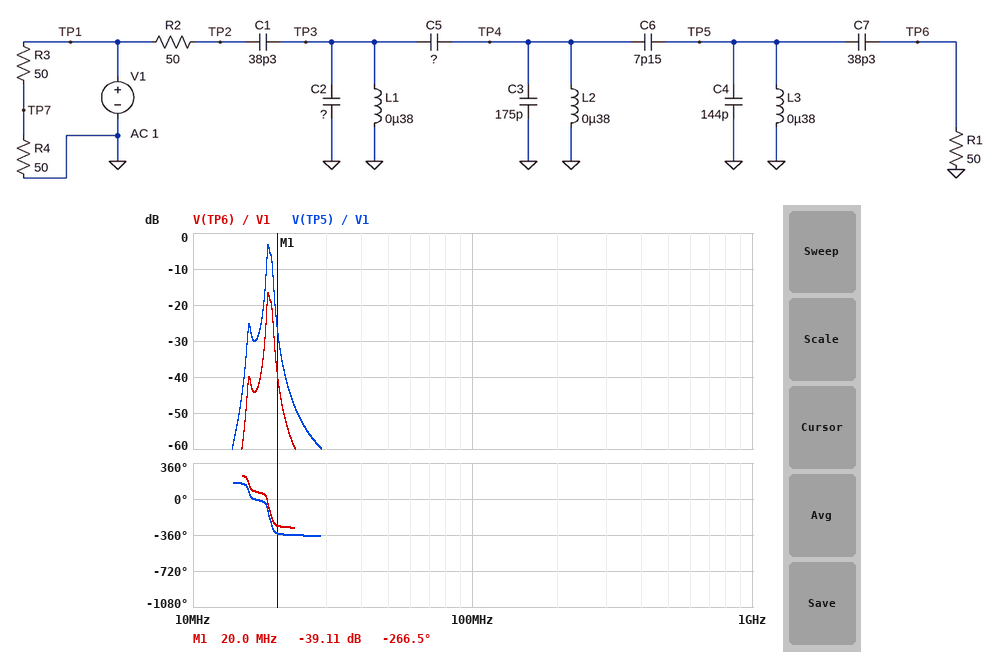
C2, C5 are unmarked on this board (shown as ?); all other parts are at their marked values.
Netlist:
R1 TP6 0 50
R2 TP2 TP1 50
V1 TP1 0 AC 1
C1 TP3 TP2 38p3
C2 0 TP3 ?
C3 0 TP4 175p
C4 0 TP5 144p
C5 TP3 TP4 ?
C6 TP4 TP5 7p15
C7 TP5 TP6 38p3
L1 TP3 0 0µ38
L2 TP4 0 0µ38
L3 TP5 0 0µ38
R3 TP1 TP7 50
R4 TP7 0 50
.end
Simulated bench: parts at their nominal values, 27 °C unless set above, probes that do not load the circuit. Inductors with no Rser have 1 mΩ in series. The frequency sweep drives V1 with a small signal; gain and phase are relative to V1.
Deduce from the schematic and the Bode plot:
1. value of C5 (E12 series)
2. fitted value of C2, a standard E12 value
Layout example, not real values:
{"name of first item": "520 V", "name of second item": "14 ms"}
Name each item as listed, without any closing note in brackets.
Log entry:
{"value of C5": "8.2 pF", "fitted value of C2, a standard E12 value": "220 pF"}
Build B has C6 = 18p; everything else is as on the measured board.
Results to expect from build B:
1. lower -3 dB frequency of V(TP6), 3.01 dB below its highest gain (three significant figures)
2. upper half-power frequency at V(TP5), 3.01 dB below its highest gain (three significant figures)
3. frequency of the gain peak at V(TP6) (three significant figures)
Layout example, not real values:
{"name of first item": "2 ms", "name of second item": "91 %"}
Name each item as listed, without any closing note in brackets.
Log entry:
{"lower -3 dB frequency of V(TP6), 3.01 dB below its highest gain": "17.4 MHz", "upper half-power frequency at V(TP5), 3.01 dB below its highest gain": "17.7 MHz", "frequency of the gain peak at V(TP6)": "17.5 MHz"}
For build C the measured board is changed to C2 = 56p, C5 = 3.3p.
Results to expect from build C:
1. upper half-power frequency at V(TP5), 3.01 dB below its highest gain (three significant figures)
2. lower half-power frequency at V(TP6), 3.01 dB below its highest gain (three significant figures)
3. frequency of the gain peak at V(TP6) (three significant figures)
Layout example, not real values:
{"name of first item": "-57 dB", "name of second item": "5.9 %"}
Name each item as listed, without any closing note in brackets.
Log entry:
{"upper half-power frequency at V(TP5), 3.01 dB below its highest gain": "19.3 MHz", "lower half-power frequency at V(TP6), 3.01 dB below its highest gain": "18.7 MHz", "frequency of the gain peak at V(TP6)": "19.2 MHz"}
